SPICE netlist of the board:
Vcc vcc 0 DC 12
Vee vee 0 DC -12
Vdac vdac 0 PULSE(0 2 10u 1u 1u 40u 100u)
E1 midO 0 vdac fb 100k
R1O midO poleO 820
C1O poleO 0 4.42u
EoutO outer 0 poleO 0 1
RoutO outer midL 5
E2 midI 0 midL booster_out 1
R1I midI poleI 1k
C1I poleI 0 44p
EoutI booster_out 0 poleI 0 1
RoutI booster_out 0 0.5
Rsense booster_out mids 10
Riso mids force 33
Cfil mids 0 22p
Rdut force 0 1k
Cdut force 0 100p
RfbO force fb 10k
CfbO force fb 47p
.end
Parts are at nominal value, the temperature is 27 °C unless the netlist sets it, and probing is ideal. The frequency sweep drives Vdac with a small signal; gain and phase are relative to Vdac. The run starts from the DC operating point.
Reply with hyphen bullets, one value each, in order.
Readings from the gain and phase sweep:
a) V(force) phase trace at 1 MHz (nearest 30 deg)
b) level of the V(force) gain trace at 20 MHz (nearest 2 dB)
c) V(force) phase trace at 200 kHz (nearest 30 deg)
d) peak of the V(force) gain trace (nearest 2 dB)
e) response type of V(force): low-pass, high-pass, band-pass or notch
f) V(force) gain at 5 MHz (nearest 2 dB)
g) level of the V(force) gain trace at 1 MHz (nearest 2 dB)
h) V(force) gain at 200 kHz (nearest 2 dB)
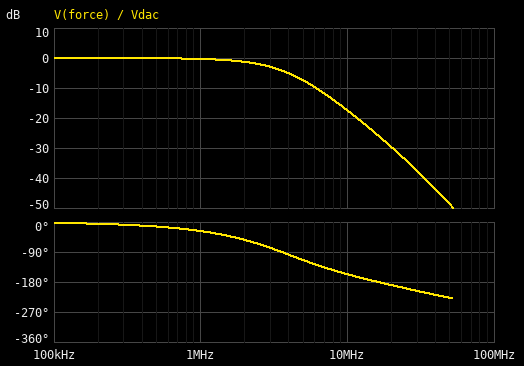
- -30 deg
- -30 dB
- 0 deg
- 0 dB
- low-pass
- -8 dB
- 0 dB
- 0 dB
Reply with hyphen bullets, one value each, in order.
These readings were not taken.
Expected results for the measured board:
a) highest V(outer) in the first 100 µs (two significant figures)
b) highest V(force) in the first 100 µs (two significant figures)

- 4.2 V
- 2.0 V
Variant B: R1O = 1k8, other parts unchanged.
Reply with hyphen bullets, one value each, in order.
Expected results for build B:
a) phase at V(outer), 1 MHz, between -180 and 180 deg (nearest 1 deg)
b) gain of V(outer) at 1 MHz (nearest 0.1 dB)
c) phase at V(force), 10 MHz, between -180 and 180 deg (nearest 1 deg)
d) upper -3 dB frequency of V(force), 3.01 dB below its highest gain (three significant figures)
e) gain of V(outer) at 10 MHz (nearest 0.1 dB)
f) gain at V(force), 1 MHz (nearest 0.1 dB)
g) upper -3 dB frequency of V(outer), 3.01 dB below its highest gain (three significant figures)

- -42 deg
- 4.0 dB
- -158 deg
- 1.14 MHz
- -13.5 dB
- -2.5 dB
- 1.17 MHz
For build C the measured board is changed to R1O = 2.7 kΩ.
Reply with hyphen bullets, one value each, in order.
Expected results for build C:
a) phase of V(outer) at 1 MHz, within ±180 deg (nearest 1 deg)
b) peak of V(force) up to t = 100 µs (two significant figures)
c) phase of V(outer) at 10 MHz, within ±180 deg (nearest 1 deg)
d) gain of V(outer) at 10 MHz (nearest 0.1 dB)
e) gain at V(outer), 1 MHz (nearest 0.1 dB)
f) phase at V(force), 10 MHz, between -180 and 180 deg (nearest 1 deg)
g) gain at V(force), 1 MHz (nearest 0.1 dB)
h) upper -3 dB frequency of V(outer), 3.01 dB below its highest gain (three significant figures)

- -55 deg
- 2.0 V
- -89 deg
- -17.2 dB
- 1.7 dB
- -159 deg
- -4.7 dB
- 723 kHz
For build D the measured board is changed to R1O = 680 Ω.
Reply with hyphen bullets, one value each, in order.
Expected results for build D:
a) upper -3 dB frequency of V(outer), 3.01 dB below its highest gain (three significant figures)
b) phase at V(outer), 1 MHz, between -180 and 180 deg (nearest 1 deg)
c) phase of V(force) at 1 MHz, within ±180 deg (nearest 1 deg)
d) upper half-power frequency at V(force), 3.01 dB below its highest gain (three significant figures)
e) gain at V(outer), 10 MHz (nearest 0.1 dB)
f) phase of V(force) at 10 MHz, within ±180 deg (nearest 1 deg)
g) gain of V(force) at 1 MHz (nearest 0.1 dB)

- 4.53 MHz
- -13 deg
- -23 deg
- 3.79 MHz
- -4.3 dB
- -156 deg
- -0.1 dB
